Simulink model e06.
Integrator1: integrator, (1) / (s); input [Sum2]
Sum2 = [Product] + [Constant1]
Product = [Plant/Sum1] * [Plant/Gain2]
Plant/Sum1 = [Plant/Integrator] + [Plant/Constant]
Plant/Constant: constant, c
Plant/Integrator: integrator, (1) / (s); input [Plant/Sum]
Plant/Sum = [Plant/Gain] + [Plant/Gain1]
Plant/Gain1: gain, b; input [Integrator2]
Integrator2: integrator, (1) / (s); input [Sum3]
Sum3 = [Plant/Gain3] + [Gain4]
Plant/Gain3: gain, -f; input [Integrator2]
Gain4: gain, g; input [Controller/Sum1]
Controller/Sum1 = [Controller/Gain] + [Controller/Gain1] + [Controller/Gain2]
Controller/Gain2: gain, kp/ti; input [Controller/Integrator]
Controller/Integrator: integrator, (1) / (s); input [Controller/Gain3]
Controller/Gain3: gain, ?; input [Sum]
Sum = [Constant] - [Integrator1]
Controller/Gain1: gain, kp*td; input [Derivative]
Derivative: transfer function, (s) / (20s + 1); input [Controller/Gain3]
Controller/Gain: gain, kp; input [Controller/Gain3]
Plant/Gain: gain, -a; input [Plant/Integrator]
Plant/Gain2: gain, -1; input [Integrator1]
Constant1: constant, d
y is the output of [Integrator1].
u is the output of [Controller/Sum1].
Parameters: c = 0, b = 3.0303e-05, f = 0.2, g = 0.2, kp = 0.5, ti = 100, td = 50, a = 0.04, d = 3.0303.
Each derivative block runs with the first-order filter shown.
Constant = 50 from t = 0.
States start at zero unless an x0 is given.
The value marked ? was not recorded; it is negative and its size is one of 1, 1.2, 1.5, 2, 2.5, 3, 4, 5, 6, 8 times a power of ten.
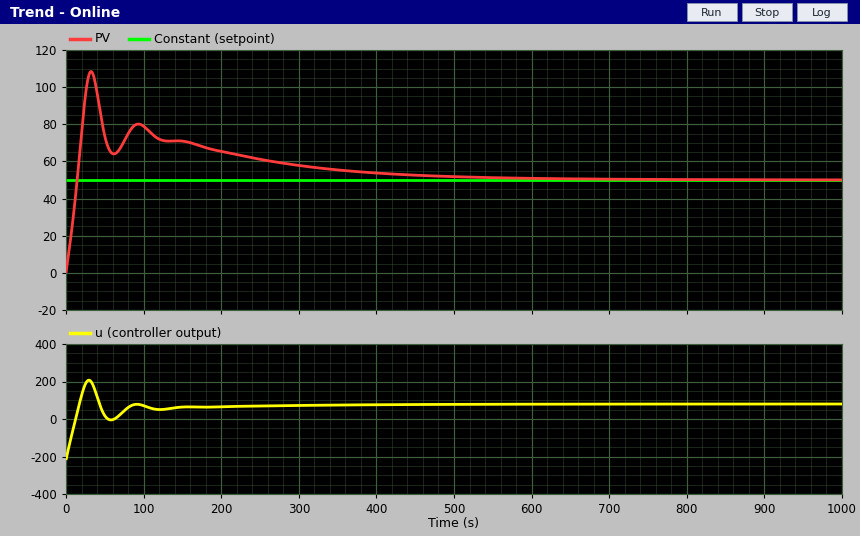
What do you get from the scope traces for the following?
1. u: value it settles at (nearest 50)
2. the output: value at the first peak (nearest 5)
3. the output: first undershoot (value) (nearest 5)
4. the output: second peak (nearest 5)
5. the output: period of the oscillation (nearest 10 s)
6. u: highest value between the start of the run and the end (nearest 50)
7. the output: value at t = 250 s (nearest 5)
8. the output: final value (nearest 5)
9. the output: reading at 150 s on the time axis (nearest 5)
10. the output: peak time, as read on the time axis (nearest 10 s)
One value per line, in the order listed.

100
110
65
80
60 s
200
60
50
70
30 s
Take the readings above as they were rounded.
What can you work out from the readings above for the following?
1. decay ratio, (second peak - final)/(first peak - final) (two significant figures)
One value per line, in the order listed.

0.50
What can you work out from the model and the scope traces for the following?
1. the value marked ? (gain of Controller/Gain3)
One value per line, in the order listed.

-2.5
